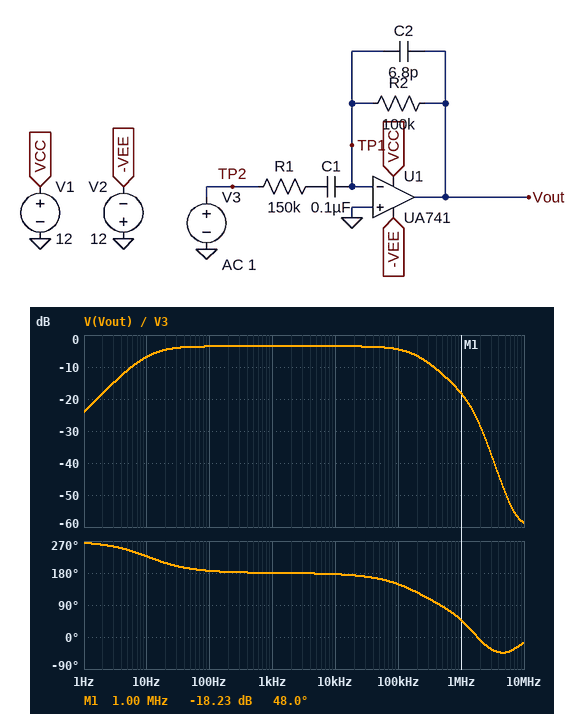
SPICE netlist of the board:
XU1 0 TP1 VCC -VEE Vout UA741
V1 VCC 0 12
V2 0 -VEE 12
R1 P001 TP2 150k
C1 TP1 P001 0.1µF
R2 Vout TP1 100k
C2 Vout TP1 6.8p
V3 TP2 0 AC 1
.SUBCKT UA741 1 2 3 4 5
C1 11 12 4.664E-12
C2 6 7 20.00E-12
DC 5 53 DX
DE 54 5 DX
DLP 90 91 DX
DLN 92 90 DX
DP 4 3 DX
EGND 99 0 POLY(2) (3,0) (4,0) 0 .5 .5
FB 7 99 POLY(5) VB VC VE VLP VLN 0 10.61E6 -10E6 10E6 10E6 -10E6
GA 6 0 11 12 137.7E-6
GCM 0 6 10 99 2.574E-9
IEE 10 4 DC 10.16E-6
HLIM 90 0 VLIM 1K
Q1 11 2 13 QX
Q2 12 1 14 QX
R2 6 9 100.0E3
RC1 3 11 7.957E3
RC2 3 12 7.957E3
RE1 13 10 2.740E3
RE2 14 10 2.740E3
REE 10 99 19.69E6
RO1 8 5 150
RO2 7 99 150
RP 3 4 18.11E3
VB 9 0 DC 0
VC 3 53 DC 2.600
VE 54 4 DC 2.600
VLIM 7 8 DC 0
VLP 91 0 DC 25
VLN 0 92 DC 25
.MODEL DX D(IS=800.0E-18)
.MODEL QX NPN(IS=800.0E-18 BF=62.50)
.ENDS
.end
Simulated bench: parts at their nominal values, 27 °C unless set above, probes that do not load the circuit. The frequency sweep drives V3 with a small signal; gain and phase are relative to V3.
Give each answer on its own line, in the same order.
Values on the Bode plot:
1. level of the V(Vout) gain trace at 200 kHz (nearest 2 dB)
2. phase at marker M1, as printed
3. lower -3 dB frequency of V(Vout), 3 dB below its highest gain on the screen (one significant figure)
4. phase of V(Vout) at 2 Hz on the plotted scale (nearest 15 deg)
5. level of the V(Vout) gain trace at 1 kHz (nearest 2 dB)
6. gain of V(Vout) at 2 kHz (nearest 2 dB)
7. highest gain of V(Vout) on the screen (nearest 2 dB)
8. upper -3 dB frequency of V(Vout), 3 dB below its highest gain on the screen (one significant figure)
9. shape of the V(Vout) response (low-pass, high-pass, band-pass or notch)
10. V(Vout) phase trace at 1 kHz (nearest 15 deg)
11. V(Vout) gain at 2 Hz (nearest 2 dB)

-6 dB
48.0 deg
10 Hz
255 deg
-4 dB
-4 dB
-4 dB
200 kHz
band-pass
180 deg
-18 dB
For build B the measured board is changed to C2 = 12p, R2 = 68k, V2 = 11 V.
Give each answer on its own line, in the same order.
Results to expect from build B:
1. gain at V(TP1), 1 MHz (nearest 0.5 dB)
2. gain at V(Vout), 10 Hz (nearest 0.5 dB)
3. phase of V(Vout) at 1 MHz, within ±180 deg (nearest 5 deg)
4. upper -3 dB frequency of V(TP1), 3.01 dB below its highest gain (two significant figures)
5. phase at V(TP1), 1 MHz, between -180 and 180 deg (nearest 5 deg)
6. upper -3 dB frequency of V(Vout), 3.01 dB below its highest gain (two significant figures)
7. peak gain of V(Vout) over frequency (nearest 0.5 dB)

-22.5 dB
-10.0 dB
45 deg
2.1 MHz
-20 deg
180 kHz
-7.0 dB
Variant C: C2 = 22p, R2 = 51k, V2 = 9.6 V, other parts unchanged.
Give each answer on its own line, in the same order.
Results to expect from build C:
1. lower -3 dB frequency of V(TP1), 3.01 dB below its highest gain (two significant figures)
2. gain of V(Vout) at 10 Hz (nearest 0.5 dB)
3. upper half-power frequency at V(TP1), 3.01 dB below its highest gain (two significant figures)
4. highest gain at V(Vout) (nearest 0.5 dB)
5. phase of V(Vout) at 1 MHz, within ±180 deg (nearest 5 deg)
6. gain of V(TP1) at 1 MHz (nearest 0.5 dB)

140 kHz
-12.5 dB
2.0 MHz
-9.5 dB
40 deg
-27.5 dB
